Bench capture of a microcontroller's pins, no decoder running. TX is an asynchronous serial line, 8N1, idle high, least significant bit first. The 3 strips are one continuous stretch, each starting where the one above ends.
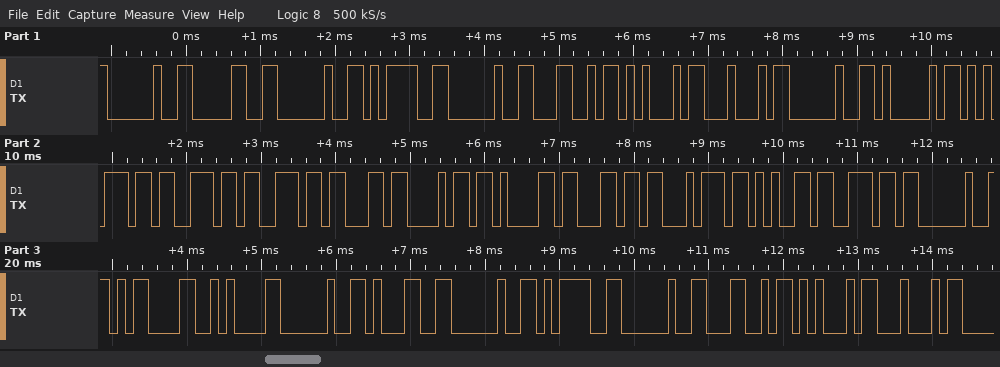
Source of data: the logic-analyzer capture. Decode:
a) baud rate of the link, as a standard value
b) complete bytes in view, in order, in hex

9600 baud
20 30 20 3D 20 4C 45 44 20 41 75 73 73 63 68 61 6C 74 65 6E 20 0D 0A 20 31 20 3D 20 4C 45 44
